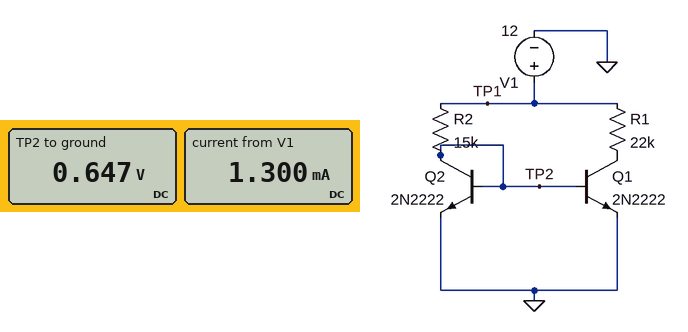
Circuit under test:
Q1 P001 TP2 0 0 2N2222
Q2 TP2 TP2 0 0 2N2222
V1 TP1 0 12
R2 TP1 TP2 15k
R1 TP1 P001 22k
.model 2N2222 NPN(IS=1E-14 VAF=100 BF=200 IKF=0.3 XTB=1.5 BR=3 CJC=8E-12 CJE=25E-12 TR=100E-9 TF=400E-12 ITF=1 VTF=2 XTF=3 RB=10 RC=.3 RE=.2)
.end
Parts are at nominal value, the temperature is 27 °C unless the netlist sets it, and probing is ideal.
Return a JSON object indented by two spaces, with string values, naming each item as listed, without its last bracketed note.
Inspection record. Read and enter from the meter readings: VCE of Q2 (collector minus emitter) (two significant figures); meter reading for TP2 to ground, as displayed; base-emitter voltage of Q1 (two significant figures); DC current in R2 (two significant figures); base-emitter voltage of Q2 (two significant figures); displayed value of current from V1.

{
  "VCE of Q2 (collector minus emitter)": "650 mV",
  "meter reading for TP2 to ground, as displayed": "0.647 V",
  "base-emitter voltage of Q1": "650 mV",
  "DC current in R2": "760 µA",
  "base-emitter voltage of Q2": "650 mV",
  "displayed value of current from V1": "1.300 mA"
}
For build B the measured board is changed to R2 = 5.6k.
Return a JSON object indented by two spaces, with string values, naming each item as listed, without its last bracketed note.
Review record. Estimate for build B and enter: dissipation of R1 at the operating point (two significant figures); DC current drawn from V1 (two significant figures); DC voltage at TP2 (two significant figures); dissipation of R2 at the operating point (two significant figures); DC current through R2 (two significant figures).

{
  "dissipation of R1 at the operating point": "6.5 mW",
  "DC current drawn from V1": "2.6 mA",
  "DC voltage at TP2": "670 mV",
  "dissipation of R2 at the operating point": "23 mW",
  "DC current through R2": "2.0 mA"
}
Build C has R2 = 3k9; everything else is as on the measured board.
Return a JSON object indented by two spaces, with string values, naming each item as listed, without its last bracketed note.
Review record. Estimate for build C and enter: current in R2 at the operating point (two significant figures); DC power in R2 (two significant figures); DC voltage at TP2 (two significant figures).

{
  "current in R2 at the operating point": "2.9 mA",
  "DC power in R2": "33 mW",
  "DC voltage at TP2": "680 mV"
}
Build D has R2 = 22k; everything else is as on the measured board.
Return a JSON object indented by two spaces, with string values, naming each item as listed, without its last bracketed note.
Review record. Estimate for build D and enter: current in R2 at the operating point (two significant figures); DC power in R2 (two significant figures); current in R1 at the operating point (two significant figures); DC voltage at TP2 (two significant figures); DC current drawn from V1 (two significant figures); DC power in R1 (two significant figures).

{
  "current in R2 at the operating point": "520 µA",
  "DC power in R2": "5.9 mW",
  "current in R1 at the operating point": "510 µA",
  "DC voltage at TP2": "640 mV",
  "DC current drawn from V1": "1.0 mA",
  "DC power in R1": "5.8 mW"
}
